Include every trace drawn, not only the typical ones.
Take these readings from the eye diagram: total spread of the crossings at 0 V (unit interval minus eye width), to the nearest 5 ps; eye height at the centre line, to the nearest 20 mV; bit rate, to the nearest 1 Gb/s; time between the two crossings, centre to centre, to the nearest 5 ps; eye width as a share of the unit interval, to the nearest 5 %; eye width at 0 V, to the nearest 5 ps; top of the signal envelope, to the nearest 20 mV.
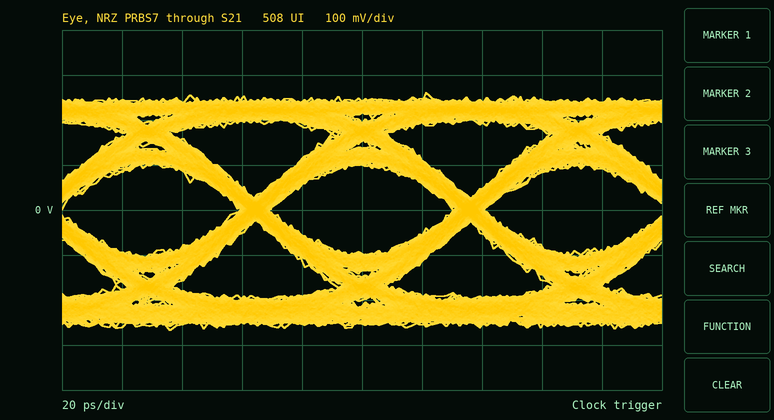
10 ps
200 mV
14 Gb/s
70 ps
85 %
60 ps
260 mV
